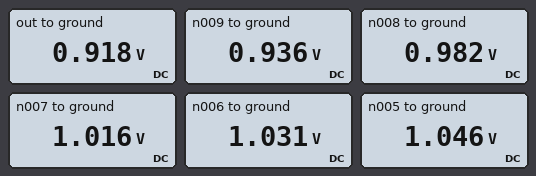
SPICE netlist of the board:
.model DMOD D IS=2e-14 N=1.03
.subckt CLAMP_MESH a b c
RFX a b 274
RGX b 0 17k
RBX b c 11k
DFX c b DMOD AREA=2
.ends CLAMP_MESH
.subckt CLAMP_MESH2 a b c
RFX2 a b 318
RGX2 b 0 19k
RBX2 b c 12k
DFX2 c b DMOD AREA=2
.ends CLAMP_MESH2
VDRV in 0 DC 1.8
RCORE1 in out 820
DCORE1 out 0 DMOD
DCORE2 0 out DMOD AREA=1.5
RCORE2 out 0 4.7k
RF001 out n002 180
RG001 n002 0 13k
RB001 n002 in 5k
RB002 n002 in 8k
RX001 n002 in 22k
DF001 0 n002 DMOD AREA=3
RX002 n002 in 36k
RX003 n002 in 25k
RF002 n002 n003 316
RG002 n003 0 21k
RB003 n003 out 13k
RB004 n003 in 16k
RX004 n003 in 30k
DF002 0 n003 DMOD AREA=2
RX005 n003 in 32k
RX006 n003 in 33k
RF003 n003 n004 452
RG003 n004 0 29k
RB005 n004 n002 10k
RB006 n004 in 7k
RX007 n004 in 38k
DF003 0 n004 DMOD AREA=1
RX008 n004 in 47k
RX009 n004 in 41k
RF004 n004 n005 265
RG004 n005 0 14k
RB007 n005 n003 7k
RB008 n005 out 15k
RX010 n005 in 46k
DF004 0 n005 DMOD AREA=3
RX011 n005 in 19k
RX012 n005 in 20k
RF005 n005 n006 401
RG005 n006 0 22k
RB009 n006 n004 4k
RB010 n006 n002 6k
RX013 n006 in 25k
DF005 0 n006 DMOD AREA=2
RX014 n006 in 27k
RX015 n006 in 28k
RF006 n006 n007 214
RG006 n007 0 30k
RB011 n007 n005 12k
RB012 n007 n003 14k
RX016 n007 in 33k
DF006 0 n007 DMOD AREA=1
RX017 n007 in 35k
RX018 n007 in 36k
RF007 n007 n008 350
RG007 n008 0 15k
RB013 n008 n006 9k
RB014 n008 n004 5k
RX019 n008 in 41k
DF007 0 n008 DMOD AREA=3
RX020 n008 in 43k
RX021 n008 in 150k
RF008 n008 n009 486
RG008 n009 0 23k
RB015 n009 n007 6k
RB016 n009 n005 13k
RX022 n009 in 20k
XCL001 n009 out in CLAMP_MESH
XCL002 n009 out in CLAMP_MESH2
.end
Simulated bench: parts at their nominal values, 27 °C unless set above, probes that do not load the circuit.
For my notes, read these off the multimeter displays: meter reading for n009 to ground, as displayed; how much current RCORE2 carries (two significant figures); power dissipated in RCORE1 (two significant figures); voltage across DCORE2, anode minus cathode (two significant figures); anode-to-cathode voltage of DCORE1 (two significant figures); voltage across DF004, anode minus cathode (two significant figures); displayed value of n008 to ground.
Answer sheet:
0.936 V
200 µA
950 µW
-920 mV
920 mV
-1.0 V
0.982 V
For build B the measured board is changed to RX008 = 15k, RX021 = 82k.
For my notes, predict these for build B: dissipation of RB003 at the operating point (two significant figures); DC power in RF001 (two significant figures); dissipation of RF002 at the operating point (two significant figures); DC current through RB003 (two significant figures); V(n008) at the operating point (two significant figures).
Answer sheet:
1.1 µW
33 µW
5.7 µW
9.2 µA
990 mV
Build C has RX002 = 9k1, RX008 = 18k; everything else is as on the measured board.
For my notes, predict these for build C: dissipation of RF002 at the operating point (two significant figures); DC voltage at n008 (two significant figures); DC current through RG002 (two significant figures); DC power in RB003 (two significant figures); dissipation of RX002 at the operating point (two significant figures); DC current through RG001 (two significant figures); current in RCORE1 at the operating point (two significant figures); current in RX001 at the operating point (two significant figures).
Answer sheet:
4.8 µW
990 mV
50 µA
1.2 µW
70 µW
77 µA
1.1 mA
36 µA
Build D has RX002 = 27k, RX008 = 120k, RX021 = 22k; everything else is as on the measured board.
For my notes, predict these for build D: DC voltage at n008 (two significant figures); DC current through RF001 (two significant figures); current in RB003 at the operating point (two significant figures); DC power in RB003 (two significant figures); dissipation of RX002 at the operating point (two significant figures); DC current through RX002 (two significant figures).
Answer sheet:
990 mV
420 µA
8.7 µA
990 nW
24 µW
30 µA
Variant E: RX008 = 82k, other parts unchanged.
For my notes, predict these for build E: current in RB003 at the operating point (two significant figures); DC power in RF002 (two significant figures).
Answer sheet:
8.5 µA
4.4 µW
